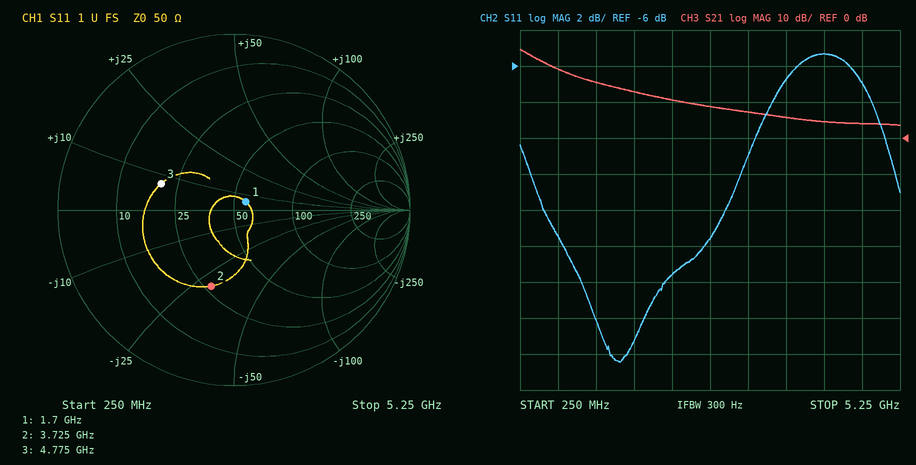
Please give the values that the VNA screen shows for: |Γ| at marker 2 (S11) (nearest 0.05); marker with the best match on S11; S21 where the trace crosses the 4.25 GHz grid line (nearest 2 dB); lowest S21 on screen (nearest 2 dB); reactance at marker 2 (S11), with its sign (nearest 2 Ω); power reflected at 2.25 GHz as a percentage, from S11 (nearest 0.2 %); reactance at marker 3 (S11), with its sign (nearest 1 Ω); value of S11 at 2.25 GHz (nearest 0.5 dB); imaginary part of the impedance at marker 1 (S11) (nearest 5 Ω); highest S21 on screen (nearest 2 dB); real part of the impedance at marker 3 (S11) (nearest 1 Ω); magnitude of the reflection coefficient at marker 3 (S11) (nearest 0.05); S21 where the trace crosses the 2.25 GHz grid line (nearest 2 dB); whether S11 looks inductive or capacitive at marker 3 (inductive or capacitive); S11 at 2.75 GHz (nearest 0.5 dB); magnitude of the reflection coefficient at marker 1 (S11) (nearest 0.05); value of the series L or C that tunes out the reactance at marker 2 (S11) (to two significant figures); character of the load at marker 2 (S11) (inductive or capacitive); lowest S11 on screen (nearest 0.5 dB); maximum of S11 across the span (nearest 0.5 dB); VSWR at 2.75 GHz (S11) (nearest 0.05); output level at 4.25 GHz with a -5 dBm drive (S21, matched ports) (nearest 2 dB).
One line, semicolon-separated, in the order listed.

0.45; marker 1; 4 dB; 4 dB; -30 Ω; 1.8 %; +7 Ω; -17.5 dB; +5 Ω; 24 dB; 20 Ω; 0.45; 10 dB; inductive; -15.5 dB; 0.10; 1.3 nH; capacitive; -22.5 dB; -5.5 dB; 1.40; 0 dBm
